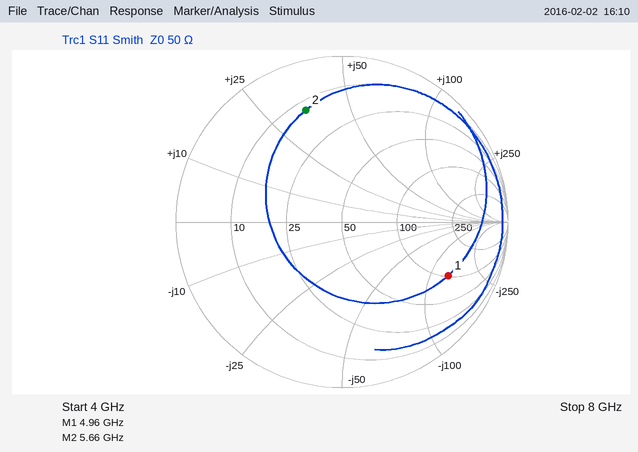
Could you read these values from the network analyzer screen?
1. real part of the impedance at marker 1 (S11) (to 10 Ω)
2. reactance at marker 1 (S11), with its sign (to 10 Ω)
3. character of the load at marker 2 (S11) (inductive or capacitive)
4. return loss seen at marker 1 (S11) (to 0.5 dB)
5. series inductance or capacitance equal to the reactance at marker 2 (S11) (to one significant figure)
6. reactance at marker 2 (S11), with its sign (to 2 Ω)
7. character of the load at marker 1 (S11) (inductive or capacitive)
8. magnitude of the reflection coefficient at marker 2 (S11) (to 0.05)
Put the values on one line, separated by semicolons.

100 Ω; -140 Ω; inductive; 3.0 dB; 1.0 nH; +34 Ω; capacitive; 0.70
